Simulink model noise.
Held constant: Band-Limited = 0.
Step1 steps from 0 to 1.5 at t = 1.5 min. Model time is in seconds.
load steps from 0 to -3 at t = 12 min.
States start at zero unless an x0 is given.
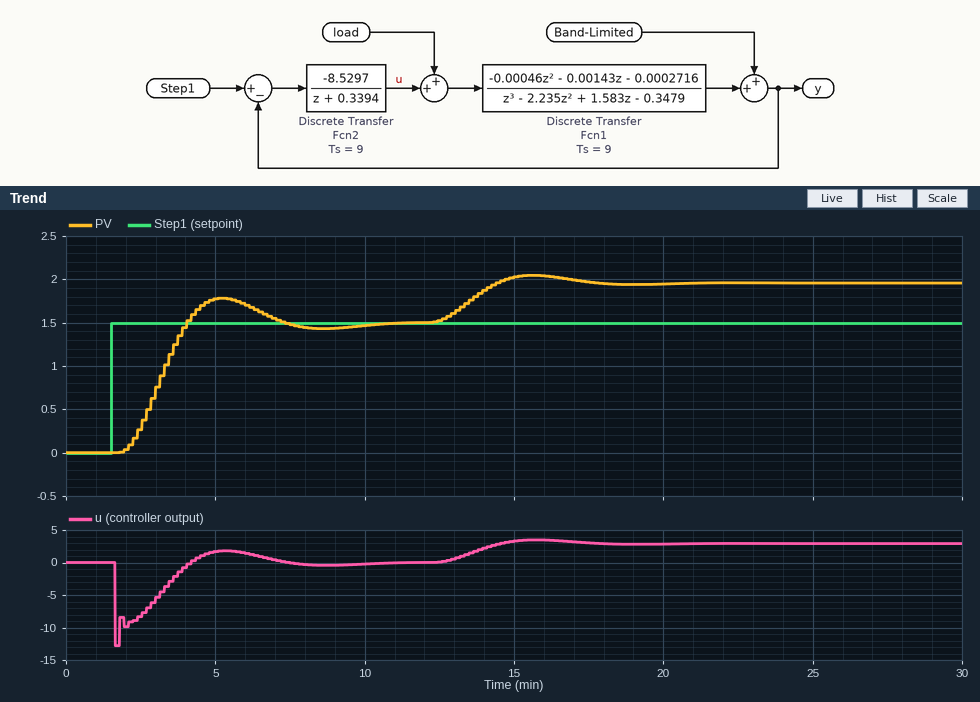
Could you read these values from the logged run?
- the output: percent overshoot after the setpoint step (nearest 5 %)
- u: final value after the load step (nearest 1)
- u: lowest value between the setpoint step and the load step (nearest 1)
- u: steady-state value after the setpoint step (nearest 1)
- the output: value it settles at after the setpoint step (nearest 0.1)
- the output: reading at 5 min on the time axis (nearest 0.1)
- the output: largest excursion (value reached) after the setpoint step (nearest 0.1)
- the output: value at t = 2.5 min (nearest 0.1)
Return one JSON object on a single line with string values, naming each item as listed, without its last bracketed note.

{"the output: percent overshoot after the setpoint step": "20 %", "u: final value after the load step": "3", "u: lowest value between the setpoint step and the load step": "-13", "u: steady-state value after the setpoint step": "0", "the output: value it settles at after the setpoint step": "1.5", "the output: reading at 5 min on the time axis": "1.8", "the output: largest excursion (value reached) after the setpoint step": "1.8", "the output: value at t = 2.5 min": "0.3"}
